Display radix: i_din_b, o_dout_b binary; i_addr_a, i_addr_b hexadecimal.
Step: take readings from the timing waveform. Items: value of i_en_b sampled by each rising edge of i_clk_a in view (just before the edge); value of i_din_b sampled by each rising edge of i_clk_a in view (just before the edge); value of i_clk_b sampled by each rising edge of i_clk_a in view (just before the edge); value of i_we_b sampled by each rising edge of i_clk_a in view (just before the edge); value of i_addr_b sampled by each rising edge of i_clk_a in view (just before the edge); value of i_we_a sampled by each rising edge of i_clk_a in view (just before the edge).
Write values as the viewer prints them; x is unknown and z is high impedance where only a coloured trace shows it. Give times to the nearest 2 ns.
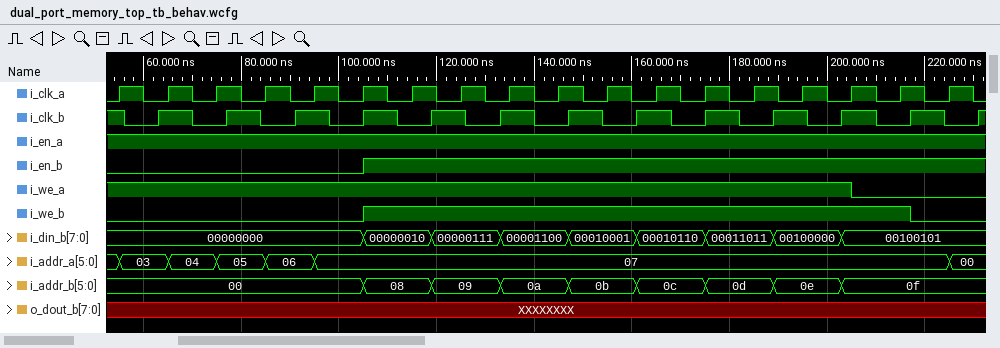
0 0 0 0 0 0 1 1 1 1 1 1 1 1 1 1 1 1
00000000, 00000000, 00000000, 00000000, 00000000, 00000000, 00000010, 00000111, 00001100, 00001100, 00010001, 00010110, 00010110, 00011011, 00100000, 00100101, 00100101, 00100101
1 1 0 0 1 0 0 1 1 0 0 1 0 0 1 1 0 0
0 0 0 0 0 0 1 1 1 1 1 1 1 1 1 1 1 0
00, 00, 00, 00, 00, 00, 08, 09, 0a, 0a, 0b, 0c, 0c, 0d, 0e, 0f, 0f, 0f
1 1 1 1 1 1 1 1 1 1 1 1 1 1 1 1 0 0
